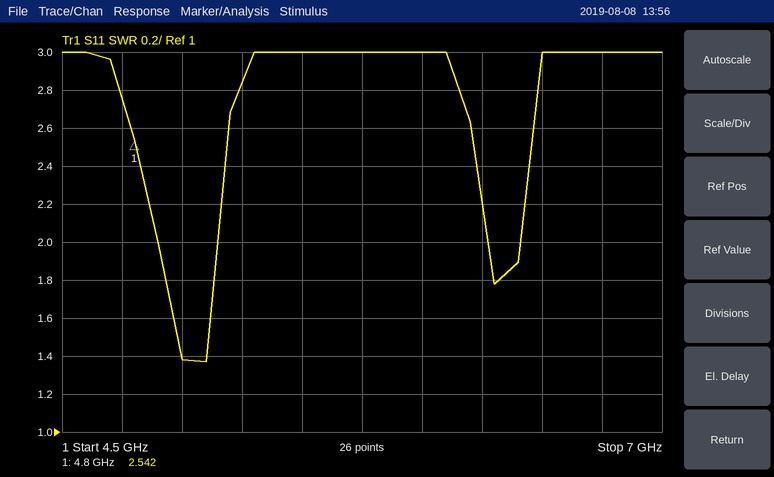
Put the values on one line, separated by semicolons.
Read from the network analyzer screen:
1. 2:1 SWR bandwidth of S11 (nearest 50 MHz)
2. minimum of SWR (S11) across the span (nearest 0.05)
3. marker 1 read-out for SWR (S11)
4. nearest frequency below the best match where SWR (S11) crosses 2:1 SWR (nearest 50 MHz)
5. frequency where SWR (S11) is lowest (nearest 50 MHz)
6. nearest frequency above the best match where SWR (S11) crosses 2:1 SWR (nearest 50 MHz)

250 MHz; 1.35; 2.542; 4.90 GHz; 5.10 GHz; 5.15 GHz
